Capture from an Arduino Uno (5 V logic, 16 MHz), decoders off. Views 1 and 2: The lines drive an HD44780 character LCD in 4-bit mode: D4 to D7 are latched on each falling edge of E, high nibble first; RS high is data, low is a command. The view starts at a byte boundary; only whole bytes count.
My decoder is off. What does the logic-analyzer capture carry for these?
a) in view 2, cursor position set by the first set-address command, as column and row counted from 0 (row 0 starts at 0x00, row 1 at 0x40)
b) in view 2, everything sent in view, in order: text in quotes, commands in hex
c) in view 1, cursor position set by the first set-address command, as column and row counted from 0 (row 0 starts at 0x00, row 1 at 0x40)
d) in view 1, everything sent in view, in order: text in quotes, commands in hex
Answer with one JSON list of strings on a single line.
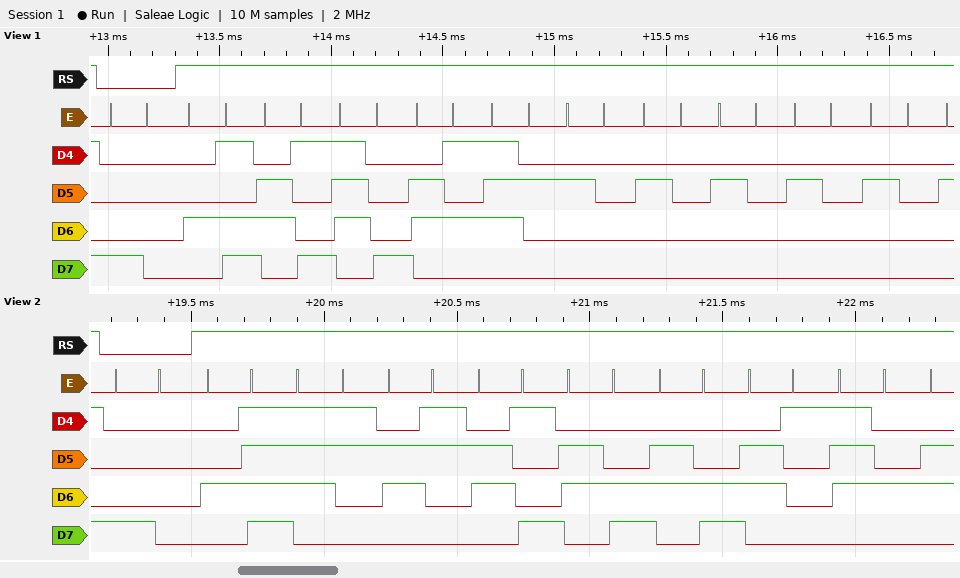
["column 0, row 0", "0x80 \"Oscillat\"", "column 0, row 0", "0x80 \"Mixer     \""]
